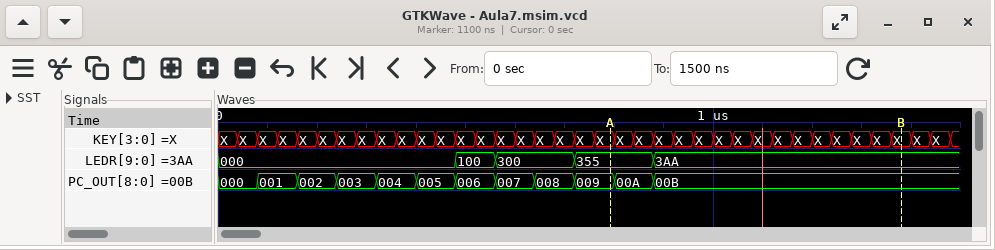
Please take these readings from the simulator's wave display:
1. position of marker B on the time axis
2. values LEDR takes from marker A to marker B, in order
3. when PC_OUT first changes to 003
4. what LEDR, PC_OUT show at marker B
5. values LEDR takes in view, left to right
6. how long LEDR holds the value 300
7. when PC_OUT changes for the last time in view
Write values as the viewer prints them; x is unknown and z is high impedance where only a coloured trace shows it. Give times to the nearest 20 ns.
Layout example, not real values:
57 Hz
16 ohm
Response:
1380 ns
355, 3AA
240 ns
LEDR=3AA, PC_OUT=00B
000, 100, 300, 355, 3AA
160 ns
880 ns
